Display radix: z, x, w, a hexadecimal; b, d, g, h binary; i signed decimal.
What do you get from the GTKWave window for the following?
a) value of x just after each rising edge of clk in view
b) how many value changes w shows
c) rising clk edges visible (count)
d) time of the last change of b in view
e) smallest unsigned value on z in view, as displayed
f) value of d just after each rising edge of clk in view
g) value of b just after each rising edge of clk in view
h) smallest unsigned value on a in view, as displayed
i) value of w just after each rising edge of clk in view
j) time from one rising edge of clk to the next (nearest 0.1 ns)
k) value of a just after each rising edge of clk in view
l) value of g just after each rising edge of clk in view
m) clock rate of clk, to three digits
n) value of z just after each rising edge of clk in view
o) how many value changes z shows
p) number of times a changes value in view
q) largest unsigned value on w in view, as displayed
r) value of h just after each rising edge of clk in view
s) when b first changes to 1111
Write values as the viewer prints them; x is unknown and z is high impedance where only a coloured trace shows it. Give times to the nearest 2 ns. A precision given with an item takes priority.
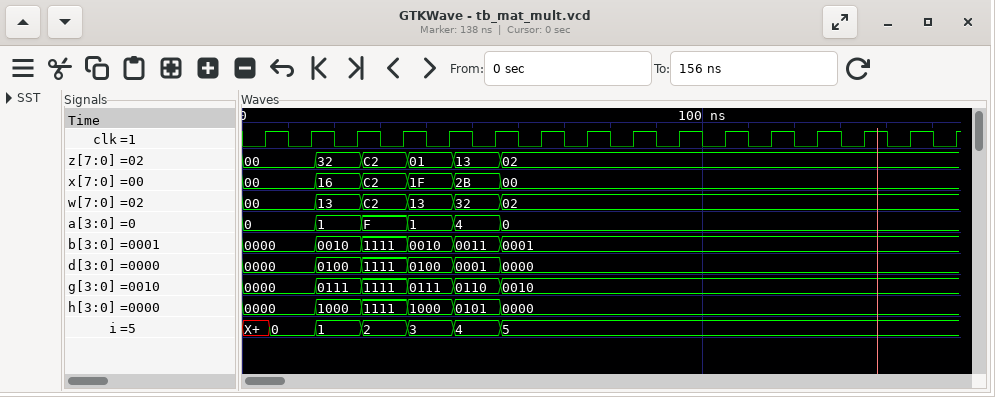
00, 00, 16, C2, 1F, 2B, 00, 00, 00, 00, 00, 00, 00, 00, 00, 00
5
16
56 ns
00
0000, 0000, 0100, 1111, 0100, 0001, 0000, 0000, 0000, 0000, 0000, 0000, 0000, 0000, 0000, 0000
0000, 0000, 0010, 1111, 0010, 0011, 0001, 0001, 0001, 0001, 0001, 0001, 0001, 0001, 0001, 0001
0
00, 00, 13, C2, 13, 32, 02, 02, 02, 02, 02, 02, 02, 02, 02, 02
10 ns
0, 0, 1, F, 1, 4, 0, 0, 0, 0, 0, 0, 0, 0, 0, 0
0000, 0000, 0111, 1111, 0111, 0110, 0010, 0010, 0010, 0010, 0010, 0010, 0010, 0010, 0010, 0010
100 MHz
00, 00, 32, C2, 01, 13, 02, 02, 02, 02, 02, 02, 02, 02, 02, 02
5
5
C2
0000, 0000, 1000, 1111, 1000, 0101, 0000, 0000, 0000, 0000, 0000, 0000, 0000, 0000, 0000, 0000
26 ns
